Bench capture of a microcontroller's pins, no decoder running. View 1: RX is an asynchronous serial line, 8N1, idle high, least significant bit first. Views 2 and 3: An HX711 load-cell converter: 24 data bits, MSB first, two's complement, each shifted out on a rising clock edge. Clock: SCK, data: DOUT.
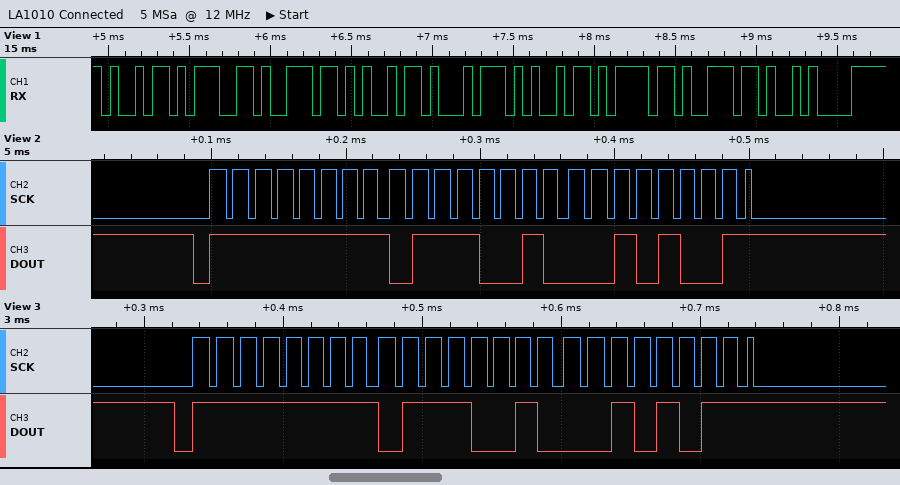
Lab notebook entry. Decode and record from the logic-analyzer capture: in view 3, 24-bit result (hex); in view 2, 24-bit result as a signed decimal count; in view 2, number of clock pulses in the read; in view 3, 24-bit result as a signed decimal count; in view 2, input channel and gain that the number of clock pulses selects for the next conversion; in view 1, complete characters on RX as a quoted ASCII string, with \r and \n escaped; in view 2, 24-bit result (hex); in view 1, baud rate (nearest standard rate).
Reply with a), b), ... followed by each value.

a) 0xFF722B
b) -36311
c) 25
d) -36309
e) channel A, gain 128
f) "ignition\n"
g) 0xFF7229
h) 19200 baud
